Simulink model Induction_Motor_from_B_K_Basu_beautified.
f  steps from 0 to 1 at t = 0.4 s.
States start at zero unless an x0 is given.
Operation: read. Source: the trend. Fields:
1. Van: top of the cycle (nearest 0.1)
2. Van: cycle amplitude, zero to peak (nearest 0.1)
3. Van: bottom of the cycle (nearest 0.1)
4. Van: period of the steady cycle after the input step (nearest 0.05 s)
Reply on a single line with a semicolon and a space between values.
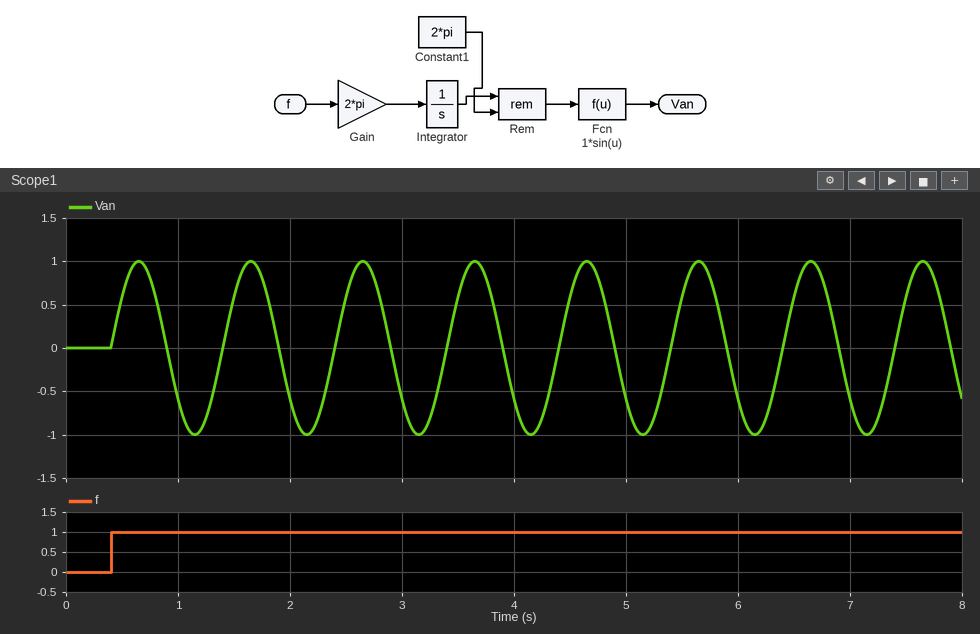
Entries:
1.0; 1.0; -1.0; 1.00 s
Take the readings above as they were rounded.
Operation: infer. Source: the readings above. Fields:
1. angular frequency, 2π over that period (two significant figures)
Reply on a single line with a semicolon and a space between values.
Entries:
6.3 rad/s
